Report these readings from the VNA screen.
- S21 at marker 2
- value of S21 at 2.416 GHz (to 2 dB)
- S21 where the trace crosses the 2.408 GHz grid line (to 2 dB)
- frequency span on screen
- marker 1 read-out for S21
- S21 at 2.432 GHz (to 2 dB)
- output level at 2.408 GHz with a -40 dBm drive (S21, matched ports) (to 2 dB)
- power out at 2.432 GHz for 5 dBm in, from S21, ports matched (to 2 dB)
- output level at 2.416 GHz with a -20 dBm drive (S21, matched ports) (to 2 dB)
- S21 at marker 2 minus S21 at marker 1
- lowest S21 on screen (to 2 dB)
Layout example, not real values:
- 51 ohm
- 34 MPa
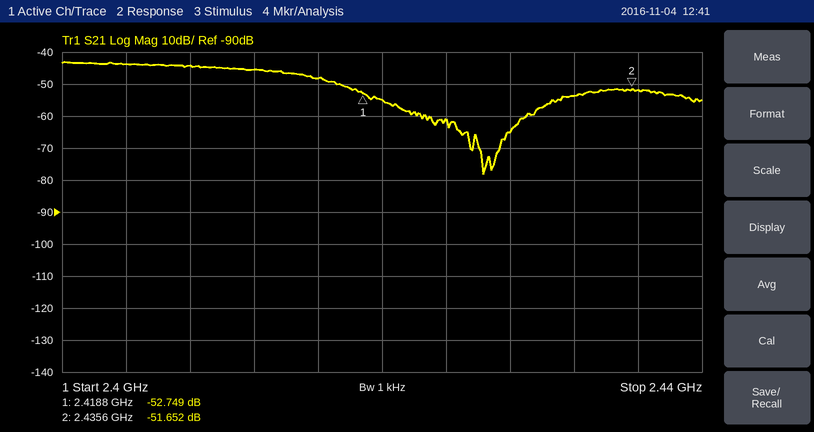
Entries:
- -51.652 dB
- -48 dB
- -44 dB
- 40 MHz
- -52.749 dB
- -54 dB
- -84 dBm
- -48 dBm
- -68 dBm
- 1.097 dB
- -78 dB
